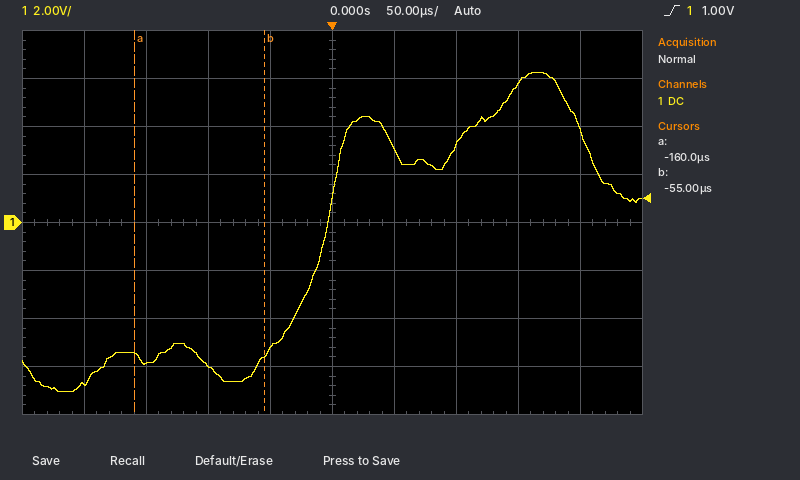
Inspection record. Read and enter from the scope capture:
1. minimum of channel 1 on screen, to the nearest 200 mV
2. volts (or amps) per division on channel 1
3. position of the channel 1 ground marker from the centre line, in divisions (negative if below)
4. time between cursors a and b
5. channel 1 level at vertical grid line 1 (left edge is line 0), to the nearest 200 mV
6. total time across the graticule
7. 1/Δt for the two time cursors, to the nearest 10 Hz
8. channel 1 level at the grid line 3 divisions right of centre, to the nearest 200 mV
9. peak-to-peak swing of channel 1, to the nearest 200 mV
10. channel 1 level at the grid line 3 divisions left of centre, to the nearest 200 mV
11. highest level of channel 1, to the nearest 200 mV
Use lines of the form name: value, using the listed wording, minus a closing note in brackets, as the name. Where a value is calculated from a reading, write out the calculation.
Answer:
minimum of channel 1 on screen, to the nearest 200 mV: -7.0 V
volts (or amps) per division on channel 1: 2 V
position of the channel 1 ground marker from the centre line, in divisions: 0.0 div
time between cursors a and b: -55 µs − (-160 µs) = 105 µs
channel 1 level at vertical grid line 1 (left edge is line 0), to the nearest 200 mV: -6.8 V
total time across the graticule: 500 µs
1/Δt for the two time cursors, to the nearest 10 Hz: 1 / 105 µs ≈ 9.52 kHz
channel 1 level at the grid line 3 divisions right of centre, to the nearest 200 mV: 5.8 V
peak-to-peak swing of channel 1, to the nearest 200 mV: 6.2 V − (-7.0 V) = 13.2 V
channel 1 level at the grid line 3 divisions left of centre, to the nearest 200 mV: -5.8 V
highest level of channel 1, to the nearest 200 mV: 6.2 V
